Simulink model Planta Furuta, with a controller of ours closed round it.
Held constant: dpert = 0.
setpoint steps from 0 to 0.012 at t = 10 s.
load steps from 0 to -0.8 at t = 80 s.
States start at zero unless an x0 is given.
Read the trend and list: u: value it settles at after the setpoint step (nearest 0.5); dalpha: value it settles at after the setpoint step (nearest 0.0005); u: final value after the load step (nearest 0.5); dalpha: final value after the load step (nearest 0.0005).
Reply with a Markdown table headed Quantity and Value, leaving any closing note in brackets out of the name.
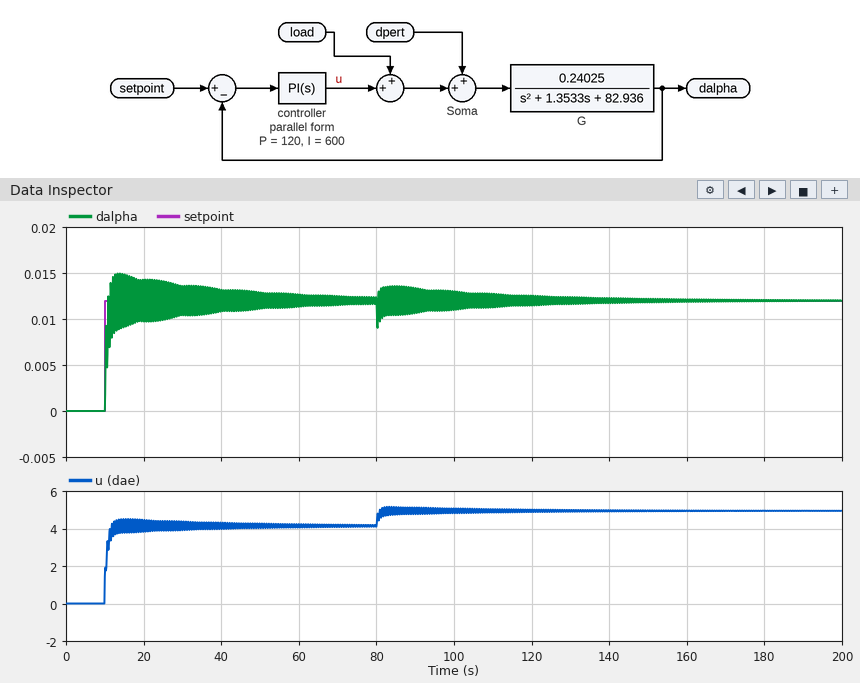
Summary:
| Quantity | Value |
|---|---|
| u: value it settles at after the setpoint step | 4.0 |
| dalpha: value it settles at after the setpoint step | 0.0120 |
| u: final value after the load step | 5.0 |
| dalpha: final value after the load step | 0.0120 |
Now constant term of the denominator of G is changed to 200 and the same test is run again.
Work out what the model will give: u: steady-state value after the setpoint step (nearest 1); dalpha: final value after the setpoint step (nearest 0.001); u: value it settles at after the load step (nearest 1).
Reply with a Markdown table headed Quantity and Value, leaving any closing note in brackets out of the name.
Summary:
| Quantity | Value |
|---|---|
| u: steady-state value after the setpoint step | 10 |
| dalpha: final value after the setpoint step | 0.012 |
| u: value it settles at after the load step | 11 |
